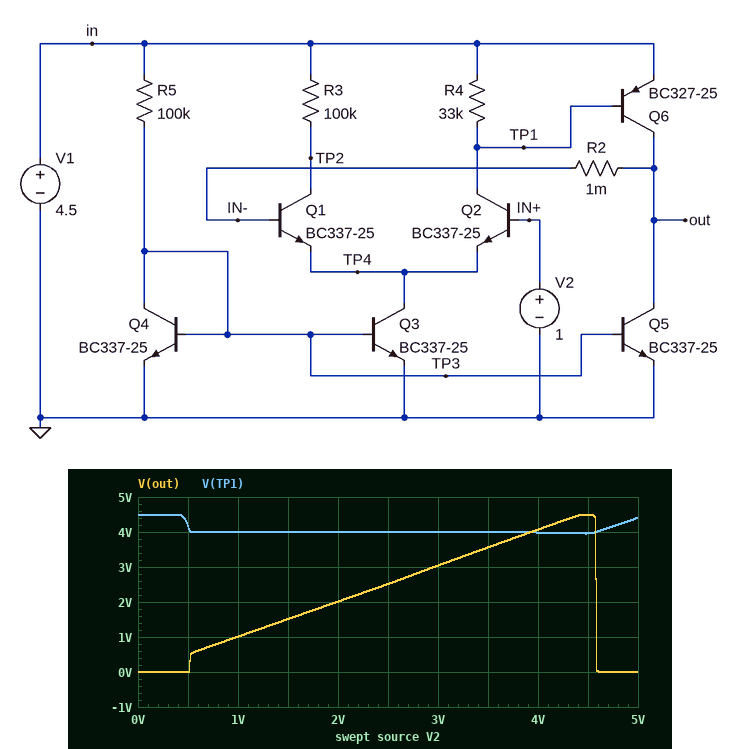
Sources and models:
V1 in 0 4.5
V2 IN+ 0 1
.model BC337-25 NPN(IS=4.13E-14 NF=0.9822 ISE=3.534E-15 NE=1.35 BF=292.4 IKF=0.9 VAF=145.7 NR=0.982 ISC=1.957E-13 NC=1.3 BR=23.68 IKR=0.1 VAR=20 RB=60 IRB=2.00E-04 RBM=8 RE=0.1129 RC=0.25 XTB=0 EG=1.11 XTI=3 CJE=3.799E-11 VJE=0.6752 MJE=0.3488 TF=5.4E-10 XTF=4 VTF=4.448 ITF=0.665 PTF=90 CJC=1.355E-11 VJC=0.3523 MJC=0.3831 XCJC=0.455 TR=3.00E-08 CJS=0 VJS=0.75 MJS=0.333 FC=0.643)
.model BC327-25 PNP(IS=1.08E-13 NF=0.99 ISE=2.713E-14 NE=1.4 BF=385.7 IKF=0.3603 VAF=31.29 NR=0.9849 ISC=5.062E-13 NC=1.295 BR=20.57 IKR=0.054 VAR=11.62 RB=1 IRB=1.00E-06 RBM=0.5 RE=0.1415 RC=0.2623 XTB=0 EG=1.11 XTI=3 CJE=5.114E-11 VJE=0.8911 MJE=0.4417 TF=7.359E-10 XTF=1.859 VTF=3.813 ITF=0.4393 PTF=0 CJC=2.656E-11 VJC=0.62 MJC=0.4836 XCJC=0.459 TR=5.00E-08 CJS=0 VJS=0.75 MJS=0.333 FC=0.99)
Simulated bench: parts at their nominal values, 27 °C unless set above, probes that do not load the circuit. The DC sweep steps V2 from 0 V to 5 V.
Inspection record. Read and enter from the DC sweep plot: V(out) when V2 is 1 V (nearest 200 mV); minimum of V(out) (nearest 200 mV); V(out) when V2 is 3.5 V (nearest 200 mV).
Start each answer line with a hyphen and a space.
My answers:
- 1.0 V
- 0 V
- 3.6 V
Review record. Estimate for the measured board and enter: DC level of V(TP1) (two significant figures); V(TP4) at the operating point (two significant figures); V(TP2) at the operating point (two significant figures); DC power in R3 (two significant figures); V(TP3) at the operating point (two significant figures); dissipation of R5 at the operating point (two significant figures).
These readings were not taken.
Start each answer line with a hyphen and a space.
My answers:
- 4.0 V
- 500 mV
- 2.1 V
- 56 µW
- 530 mV
- 160 µW
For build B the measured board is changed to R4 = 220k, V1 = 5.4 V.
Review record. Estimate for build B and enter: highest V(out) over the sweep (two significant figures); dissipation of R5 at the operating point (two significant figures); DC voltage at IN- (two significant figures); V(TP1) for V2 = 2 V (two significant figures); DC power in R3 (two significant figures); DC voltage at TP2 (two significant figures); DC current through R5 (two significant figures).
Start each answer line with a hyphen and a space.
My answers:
- 5.1 V
- 240 µW
- 1.1 V
- 4.9 V
- 210 µW
- 850 mV
- 49 µA
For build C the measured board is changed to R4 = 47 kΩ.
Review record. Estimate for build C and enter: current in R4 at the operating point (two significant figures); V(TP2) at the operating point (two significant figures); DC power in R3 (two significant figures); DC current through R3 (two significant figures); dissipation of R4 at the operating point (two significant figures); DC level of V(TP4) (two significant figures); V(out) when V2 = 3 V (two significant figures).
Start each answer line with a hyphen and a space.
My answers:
- 11 µA
- 1.7 V
- 80 µW
- 28 µA
- 5.4 µW
- 510 mV
- 3.1 V
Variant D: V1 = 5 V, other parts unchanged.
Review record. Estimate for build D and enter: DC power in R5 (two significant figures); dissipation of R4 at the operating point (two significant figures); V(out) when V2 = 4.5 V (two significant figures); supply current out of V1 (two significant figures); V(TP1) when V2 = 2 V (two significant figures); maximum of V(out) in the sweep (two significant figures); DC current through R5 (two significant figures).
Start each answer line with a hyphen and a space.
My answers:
- 200 µW
- 7.8 µW
- 4.6 V
- 130 µA
- 4.5 V
- 5.0 V
- 45 µA
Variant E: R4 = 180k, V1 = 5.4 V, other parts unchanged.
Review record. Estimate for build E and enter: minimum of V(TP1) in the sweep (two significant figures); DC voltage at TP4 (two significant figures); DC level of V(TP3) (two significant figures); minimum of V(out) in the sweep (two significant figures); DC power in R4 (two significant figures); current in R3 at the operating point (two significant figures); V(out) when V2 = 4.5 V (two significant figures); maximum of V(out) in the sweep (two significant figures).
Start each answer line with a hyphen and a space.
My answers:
- 4.9 V
- 540 mV
- 530 mV
- 1.9 mV
- 1.4 µW
- 45 µA
- 4.6 V
- 5.1 V
